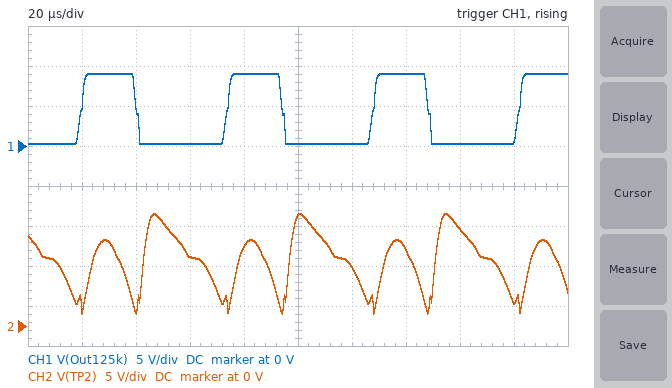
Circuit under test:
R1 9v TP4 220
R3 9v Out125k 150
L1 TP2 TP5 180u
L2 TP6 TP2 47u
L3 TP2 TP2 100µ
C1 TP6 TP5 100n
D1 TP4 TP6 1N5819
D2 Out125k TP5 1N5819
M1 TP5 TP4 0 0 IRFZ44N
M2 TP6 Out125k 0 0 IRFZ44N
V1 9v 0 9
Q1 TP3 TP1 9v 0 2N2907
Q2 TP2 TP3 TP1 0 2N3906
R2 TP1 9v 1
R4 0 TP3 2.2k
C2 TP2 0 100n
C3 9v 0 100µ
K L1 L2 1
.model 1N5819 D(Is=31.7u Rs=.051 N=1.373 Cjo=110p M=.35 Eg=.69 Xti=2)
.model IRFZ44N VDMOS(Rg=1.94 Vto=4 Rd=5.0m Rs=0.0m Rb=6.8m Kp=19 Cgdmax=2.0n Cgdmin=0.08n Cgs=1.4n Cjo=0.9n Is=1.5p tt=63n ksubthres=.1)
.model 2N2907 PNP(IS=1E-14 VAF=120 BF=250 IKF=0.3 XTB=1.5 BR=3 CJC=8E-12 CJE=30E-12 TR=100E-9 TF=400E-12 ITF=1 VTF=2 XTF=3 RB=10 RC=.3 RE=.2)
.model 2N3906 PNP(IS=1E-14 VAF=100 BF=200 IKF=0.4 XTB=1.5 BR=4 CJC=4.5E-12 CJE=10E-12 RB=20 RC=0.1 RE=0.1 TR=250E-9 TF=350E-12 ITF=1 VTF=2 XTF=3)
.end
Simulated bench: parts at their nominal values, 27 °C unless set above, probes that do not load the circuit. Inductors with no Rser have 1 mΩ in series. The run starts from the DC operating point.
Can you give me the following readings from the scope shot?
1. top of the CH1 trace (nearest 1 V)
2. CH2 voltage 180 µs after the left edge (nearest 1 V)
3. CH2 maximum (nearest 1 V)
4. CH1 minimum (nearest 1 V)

9 V
3 V
14 V
0 V
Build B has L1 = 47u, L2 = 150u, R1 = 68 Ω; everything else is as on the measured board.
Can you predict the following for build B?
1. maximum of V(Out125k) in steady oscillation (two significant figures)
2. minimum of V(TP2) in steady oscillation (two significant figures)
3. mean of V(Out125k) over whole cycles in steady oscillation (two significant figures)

9.0 V
1.5 V
5.1 V
